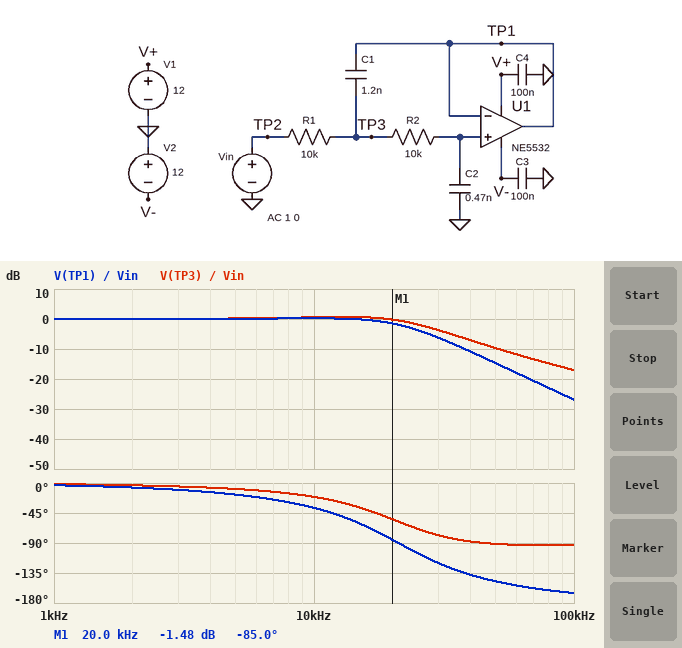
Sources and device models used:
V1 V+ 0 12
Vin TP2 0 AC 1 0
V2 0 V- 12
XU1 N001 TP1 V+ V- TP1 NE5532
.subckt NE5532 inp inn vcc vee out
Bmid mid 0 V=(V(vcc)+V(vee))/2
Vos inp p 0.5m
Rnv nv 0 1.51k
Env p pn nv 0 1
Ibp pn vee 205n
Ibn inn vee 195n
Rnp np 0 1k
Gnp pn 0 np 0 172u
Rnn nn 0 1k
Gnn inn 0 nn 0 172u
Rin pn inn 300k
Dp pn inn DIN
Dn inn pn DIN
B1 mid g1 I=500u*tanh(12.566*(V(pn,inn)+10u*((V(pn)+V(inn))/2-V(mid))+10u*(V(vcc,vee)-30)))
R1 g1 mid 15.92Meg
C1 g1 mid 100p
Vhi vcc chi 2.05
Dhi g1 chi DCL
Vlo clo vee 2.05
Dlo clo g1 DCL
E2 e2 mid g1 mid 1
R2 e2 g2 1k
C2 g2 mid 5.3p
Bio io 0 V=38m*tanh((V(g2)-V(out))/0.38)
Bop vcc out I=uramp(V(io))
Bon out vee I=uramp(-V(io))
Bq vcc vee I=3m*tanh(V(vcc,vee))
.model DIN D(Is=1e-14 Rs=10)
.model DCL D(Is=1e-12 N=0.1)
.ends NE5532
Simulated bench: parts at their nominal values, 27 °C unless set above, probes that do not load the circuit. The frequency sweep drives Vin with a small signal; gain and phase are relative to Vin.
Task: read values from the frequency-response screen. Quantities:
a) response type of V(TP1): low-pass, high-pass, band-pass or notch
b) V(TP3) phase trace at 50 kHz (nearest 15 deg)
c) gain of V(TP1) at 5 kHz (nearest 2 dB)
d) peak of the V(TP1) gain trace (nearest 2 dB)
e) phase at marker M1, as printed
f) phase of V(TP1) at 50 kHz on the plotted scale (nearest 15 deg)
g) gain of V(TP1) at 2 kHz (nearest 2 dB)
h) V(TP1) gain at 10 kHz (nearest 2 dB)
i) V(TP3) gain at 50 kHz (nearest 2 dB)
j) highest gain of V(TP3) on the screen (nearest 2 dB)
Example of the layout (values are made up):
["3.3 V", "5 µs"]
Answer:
["low-pass", "-90 deg", "0 dB", "0 dB", "-85.0 deg", "-150 deg", "0 dB", "0 dB", "-10 dB", "0 dB"]
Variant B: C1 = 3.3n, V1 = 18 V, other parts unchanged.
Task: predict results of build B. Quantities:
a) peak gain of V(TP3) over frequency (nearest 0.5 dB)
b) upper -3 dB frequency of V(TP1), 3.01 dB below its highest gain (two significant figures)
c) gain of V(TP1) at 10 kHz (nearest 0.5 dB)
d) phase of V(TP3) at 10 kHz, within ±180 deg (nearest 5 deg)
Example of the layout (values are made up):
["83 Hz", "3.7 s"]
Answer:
["3.5 dB", "15 kHz", "3.0 dB", "-40 deg"]
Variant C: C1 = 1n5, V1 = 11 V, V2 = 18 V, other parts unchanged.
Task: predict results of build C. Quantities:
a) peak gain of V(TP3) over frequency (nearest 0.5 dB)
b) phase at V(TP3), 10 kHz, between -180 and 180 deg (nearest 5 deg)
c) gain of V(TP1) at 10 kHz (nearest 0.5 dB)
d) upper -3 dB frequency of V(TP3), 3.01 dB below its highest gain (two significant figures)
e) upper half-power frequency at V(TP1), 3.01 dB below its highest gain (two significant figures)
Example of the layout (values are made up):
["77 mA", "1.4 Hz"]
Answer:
["1.0 dB", "-25 deg", "0.5 dB", "24 kHz", "22 kHz"]
